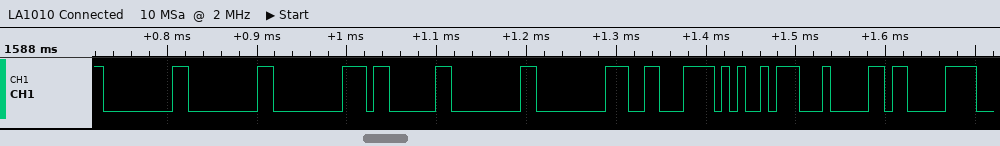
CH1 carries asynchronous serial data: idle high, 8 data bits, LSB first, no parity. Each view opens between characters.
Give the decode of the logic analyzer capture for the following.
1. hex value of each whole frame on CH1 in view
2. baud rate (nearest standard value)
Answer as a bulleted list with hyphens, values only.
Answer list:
- 00, 00, 00, 03, 00, 00, C6, A5, 04, 83
- 115200 baud
